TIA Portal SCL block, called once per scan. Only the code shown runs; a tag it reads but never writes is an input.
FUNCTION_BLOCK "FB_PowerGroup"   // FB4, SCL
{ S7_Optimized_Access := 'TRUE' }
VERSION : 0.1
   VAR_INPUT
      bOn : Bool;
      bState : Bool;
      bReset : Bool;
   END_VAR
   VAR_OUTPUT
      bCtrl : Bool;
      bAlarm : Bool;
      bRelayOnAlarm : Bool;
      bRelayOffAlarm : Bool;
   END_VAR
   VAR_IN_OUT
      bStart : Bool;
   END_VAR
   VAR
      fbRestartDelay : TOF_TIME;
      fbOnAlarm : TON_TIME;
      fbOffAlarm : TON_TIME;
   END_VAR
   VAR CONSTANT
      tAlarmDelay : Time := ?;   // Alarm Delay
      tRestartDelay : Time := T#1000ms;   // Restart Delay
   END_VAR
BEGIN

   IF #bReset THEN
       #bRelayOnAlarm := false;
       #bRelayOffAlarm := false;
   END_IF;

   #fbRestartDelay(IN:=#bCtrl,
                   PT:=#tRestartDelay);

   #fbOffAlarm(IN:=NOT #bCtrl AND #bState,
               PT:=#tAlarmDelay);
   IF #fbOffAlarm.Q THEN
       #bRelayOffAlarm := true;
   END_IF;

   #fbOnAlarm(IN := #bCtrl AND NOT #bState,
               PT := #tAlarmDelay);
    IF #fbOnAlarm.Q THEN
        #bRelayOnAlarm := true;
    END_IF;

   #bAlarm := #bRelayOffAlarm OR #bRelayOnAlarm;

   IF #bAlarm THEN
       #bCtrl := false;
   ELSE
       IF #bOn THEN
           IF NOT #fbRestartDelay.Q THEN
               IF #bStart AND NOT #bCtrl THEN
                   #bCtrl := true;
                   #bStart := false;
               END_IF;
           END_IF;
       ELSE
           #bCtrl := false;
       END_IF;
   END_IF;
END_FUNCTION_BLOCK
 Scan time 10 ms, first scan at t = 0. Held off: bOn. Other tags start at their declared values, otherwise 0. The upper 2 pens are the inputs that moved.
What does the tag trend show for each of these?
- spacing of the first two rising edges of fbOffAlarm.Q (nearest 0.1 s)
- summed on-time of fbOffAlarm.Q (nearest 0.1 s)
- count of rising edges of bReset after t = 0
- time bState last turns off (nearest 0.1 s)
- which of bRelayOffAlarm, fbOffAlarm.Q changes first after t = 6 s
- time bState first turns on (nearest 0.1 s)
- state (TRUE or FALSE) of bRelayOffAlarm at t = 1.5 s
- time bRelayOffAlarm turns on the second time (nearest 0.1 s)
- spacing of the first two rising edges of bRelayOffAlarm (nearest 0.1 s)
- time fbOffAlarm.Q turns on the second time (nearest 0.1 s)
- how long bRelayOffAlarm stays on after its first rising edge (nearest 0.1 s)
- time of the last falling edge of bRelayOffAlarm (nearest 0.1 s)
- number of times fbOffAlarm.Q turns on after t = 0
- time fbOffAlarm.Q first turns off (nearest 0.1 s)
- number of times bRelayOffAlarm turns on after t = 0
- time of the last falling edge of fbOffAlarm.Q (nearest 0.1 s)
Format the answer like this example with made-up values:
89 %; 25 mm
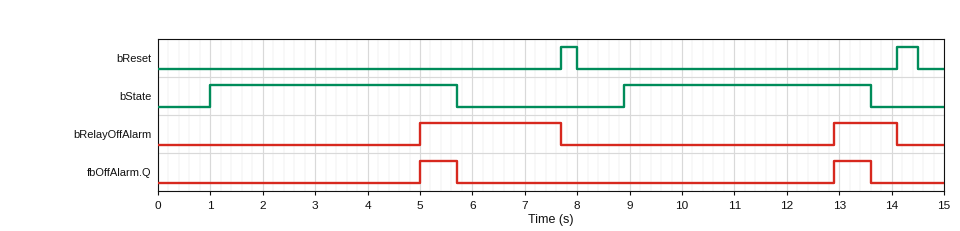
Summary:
7.9 s; 1.4 s; 2; 13.6 s; bRelayOffAlarm; 1.0 s; FALSE; 12.9 s; 7.9 s; 12.9 s; 2.7 s; 14.1 s; 2; 5.7 s; 2; 13.6 s
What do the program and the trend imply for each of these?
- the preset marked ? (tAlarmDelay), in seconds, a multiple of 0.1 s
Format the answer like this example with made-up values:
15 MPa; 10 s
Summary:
4.0 s
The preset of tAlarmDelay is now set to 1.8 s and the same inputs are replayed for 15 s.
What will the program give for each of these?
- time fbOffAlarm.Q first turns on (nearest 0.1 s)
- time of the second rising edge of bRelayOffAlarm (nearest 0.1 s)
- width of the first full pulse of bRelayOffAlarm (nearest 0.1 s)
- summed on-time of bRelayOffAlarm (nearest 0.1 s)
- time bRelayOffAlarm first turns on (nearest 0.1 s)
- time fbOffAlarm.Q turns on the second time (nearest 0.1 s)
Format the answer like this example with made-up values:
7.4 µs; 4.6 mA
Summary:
2.8 s; 10.7 s; 4.9 s; 8.3 s; 2.8 s; 10.7 s
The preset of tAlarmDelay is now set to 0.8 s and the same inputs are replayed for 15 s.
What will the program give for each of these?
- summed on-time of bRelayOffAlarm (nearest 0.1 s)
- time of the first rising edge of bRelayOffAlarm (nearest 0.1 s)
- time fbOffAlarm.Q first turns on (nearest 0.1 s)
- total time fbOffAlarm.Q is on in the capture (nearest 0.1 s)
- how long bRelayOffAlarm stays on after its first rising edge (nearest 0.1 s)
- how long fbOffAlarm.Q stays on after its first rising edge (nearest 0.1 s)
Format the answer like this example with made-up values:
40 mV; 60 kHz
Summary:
10.3 s; 1.8 s; 1.8 s; 7.8 s; 5.9 s; 3.9 s
